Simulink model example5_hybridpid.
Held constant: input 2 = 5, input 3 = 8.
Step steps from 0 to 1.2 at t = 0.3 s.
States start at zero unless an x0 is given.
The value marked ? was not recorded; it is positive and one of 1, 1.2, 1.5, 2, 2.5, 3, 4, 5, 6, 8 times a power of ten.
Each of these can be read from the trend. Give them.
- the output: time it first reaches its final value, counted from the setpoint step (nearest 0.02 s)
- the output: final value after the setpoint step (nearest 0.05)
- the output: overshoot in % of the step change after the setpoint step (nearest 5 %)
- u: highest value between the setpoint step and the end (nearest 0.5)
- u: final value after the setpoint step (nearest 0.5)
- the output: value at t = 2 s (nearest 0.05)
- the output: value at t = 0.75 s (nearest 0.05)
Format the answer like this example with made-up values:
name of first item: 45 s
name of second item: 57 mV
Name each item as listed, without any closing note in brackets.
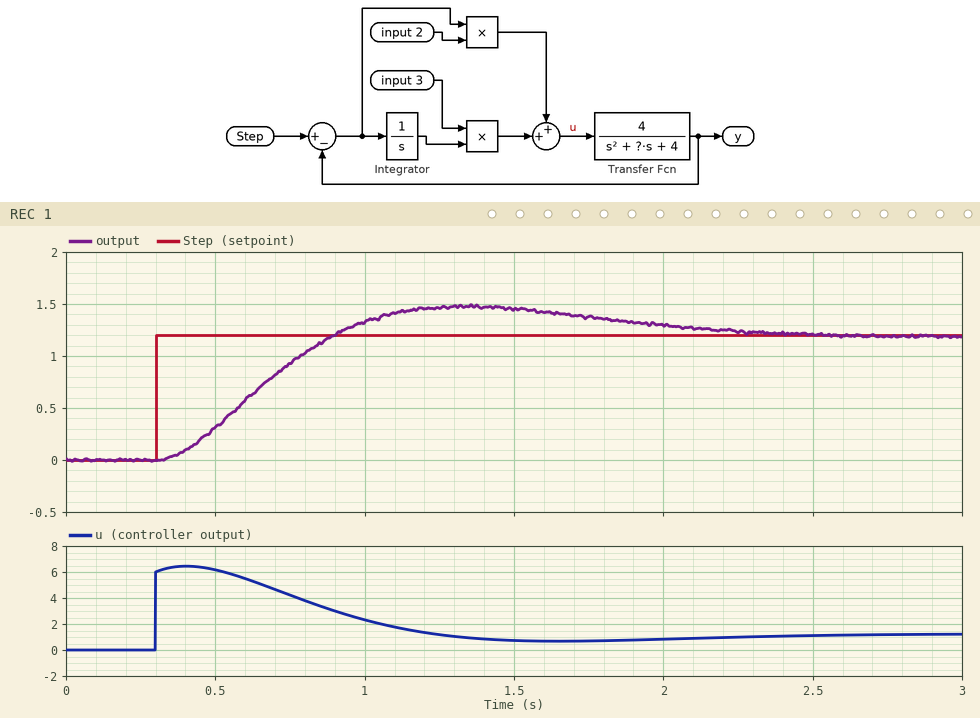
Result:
the output: time it first reaches its final value, counted from the setpoint step: 0.60 s
the output: final value after the setpoint step: 1.20
the output: overshoot in % of the step change after the setpoint step: 25 %
u: highest value between the setpoint step and the end: 6.5
u: final value after the setpoint step: 1.0
the output: value at t = 2 s: 1.30
the output: value at t = 0.75 s: 0.95
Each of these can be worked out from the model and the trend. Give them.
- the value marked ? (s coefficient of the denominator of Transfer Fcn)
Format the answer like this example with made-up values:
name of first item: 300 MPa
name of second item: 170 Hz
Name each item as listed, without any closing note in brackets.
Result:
the value marked ?: 8
